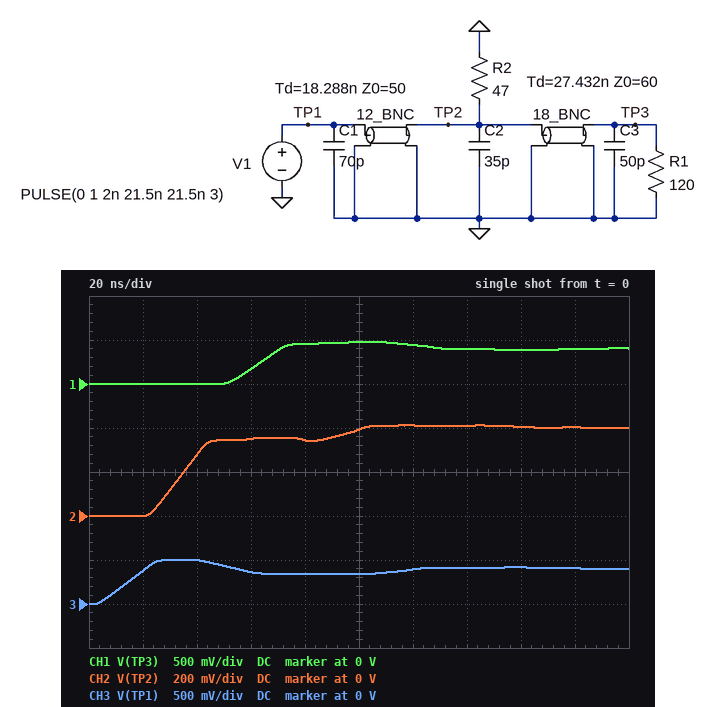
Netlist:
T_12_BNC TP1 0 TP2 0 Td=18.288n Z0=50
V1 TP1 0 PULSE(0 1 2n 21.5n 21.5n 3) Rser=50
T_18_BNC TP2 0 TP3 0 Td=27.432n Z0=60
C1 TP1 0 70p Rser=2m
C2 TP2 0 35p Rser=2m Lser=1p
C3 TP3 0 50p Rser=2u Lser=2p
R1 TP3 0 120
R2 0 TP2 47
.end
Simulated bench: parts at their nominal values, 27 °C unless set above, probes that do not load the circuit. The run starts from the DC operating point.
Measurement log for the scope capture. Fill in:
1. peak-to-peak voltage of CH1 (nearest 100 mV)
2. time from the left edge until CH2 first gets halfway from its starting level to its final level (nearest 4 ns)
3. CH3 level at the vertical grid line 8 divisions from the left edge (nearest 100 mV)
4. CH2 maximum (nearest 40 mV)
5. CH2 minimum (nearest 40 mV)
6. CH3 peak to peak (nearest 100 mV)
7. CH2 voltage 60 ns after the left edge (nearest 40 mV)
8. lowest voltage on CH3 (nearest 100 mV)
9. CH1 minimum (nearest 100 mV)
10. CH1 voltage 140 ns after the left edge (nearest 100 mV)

500 mV
36 ns
400 mV
400 mV
0 V
500 mV
360 mV
0 V
0 V
400 mV
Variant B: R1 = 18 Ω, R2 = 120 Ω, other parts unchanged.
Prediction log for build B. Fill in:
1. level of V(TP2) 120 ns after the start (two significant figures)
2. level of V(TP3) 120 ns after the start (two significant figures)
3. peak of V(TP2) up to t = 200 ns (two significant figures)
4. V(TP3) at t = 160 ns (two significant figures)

280 mV
230 mV
450 mV
240 mV
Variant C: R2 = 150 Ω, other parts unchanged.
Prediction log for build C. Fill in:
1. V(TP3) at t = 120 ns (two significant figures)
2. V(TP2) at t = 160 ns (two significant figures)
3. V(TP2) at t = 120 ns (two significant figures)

600 mV
570 mV
580 mV
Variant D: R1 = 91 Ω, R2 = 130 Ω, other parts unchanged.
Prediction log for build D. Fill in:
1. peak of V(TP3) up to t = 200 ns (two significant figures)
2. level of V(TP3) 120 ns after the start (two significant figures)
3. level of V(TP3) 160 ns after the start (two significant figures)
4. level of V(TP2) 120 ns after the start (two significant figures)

550 mV
540 mV
510 mV
520 mV
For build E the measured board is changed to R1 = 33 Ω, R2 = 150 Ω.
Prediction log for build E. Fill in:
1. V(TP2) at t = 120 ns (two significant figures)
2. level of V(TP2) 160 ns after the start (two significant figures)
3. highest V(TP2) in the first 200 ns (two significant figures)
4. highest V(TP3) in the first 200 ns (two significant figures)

370 mV
350 mV
470 mV
360 mV
